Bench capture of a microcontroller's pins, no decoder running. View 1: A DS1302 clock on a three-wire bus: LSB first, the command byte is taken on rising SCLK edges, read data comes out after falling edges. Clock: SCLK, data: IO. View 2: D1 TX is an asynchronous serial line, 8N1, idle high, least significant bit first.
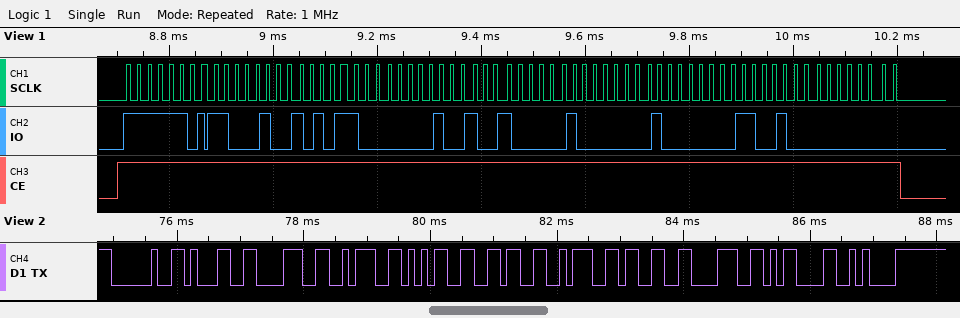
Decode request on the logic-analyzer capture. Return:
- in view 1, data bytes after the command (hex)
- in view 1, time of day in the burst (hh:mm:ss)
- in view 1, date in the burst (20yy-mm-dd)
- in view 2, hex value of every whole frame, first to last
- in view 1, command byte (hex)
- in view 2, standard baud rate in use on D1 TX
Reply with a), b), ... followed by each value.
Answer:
a) 23 35 20 09 02 02 26 00
b) 20:35:23
c) 2026-02-09
d) 20 31 38 3A 35 36 3A 33 38 0D 0A
e) 0xBF
f) 9600 baud
